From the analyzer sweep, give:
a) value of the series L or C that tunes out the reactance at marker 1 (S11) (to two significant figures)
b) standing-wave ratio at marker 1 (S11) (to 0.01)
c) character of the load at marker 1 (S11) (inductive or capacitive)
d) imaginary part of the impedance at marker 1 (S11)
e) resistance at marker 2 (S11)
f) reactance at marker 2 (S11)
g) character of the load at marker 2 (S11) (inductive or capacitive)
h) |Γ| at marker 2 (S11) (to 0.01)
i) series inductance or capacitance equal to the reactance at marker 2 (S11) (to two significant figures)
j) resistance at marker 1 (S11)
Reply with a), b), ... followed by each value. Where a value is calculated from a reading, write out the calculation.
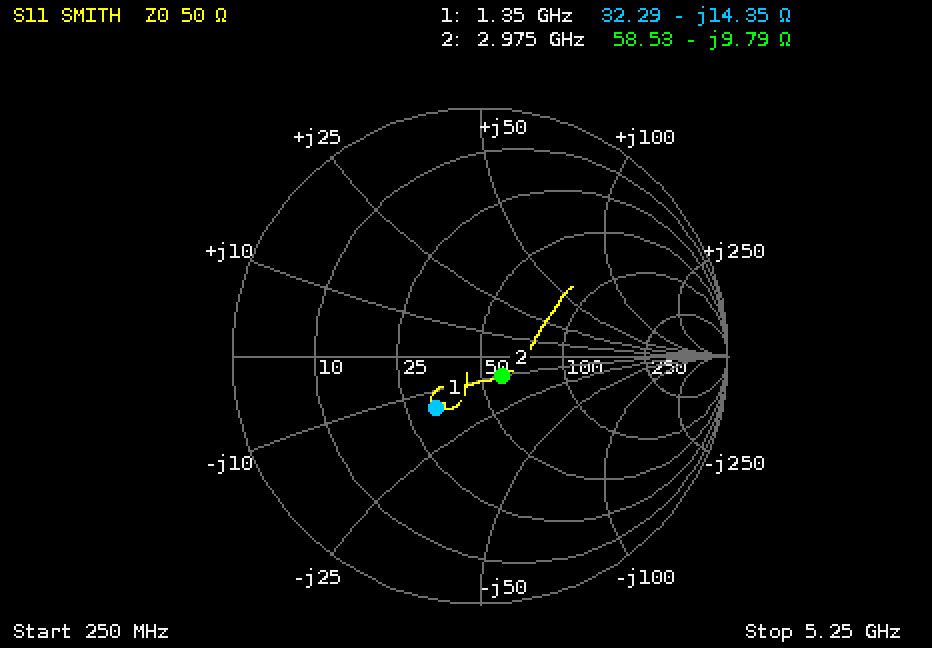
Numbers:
a) L = 14.35 Ω/(2π × 1.35 GHz) ≈ 1.7 nH
b) 1.75
c) capacitive
d) -14.35 Ω
e) 58.53 Ω
f) -9.79 Ω
g) capacitive
h) 0.12
i) C = 1/(2π × 2.975 GHz × 9.79 Ω) ≈ 5.5 pF
j) 32.29 Ω
